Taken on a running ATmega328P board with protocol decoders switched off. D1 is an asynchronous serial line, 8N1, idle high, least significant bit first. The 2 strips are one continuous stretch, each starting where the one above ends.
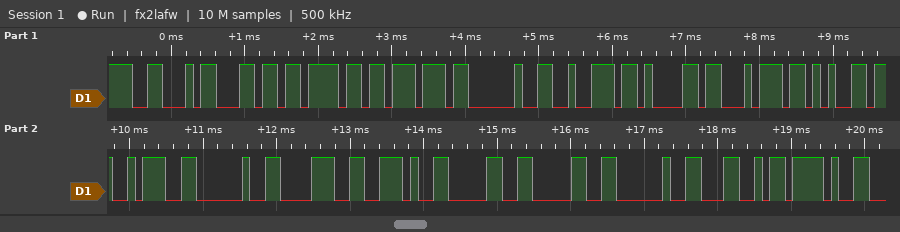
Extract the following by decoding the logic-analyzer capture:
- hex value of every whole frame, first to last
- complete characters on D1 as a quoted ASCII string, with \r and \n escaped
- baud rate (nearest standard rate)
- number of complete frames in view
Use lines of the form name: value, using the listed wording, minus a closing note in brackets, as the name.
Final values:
hex value of every whole frame, first to last: 0x46 0x6C 0x6F 0x77 0x20 0x72 0x61 0x74 0x65 0x3A 0x20 0x38 0x2E 0x30 0x30 0x20 0x4C 0x2F
complete characters on D1 as a quoted ASCII string, with \r and \n escaped: "Flow rate: 8.00 L/"
baud rate: 9600 baud
number of complete frames in view: 18
